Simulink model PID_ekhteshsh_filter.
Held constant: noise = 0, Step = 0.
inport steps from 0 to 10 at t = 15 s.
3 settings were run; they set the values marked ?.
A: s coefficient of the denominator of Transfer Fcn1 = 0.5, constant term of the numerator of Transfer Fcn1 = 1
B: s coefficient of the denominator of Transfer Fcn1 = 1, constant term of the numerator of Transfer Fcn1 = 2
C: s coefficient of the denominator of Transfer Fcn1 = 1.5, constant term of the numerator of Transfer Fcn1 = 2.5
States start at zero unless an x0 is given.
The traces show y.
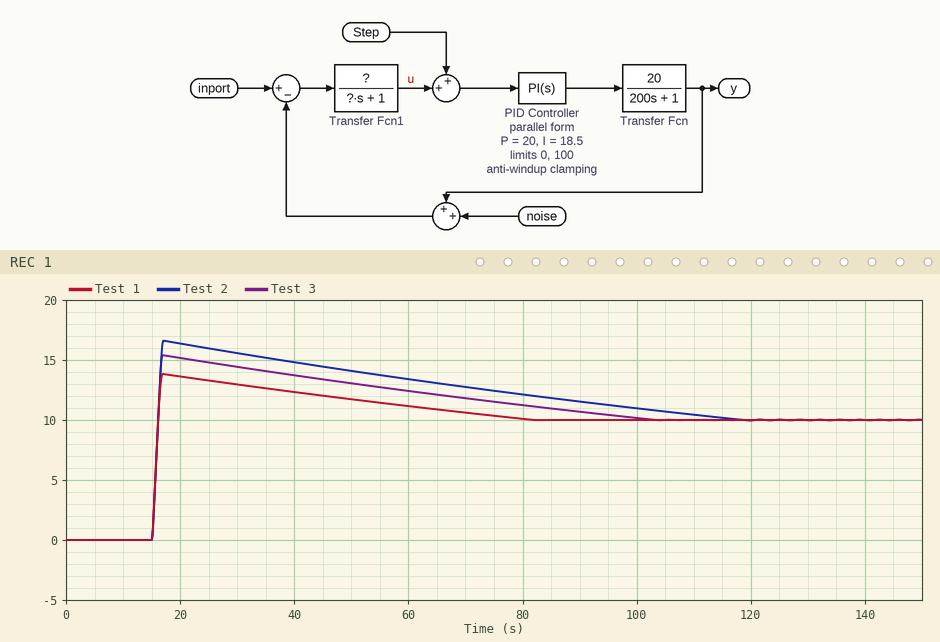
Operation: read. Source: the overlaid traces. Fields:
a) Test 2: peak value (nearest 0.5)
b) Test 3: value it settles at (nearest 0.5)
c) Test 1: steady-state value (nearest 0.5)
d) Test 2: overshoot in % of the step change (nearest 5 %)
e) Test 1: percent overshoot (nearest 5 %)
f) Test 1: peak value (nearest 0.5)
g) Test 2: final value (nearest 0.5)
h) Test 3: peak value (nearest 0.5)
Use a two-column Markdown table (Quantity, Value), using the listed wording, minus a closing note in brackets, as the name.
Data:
| Quantity | Value |
|---|---|
| Test 2: peak value | 16.5 |
| Test 3: value it settles at | 10.0 |
| Test 1: steady-state value | 10.0 |
| Test 2: overshoot in % of the step change | 65 % |
| Test 1: percent overshoot | 40 % |
| Test 1: peak value | 14.0 |
| Test 2: final value | 10.0 |
| Test 3: peak value | 15.5 |
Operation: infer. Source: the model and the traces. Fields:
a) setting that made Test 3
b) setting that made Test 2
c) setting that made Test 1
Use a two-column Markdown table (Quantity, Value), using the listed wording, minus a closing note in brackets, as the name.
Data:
| Quantity | Value |
|---|---|
| setting that made Test 3 | B |
| setting that made Test 2 | C |
| setting that made Test 1 | A |
